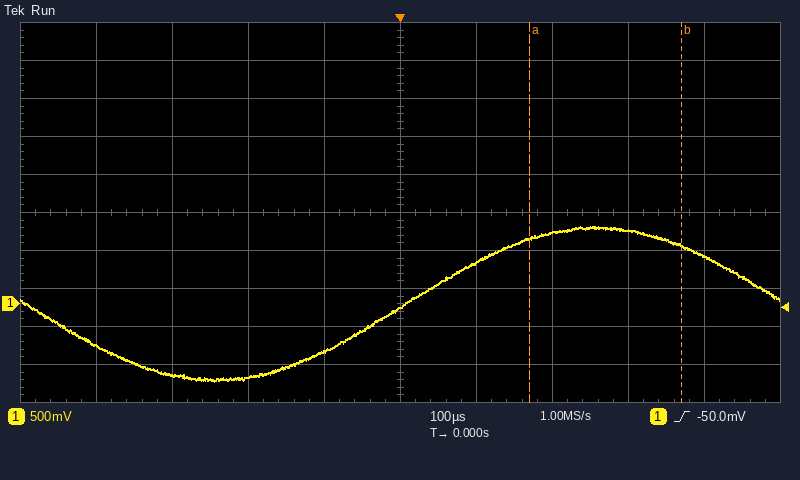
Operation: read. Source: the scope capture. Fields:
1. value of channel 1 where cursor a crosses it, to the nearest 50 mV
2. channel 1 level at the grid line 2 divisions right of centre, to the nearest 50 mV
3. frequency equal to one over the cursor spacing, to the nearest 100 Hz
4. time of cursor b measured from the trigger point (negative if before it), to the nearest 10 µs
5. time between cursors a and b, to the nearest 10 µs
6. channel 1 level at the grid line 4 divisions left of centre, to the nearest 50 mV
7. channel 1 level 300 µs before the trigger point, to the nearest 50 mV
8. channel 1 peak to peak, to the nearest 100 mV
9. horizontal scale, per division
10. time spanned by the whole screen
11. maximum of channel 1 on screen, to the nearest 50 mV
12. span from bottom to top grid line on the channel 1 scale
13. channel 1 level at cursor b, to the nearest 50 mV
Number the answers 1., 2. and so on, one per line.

1. 850 mV
2. 950 mV
3. 5.0 kHz
4. +370 µs
5. 200 µs
6. -550 mV
7. -950 mV
8. 2.00 V
9. 100 µs
10. 1 ms
11. 1.00 V
12. 5 V
13. 750 mV
